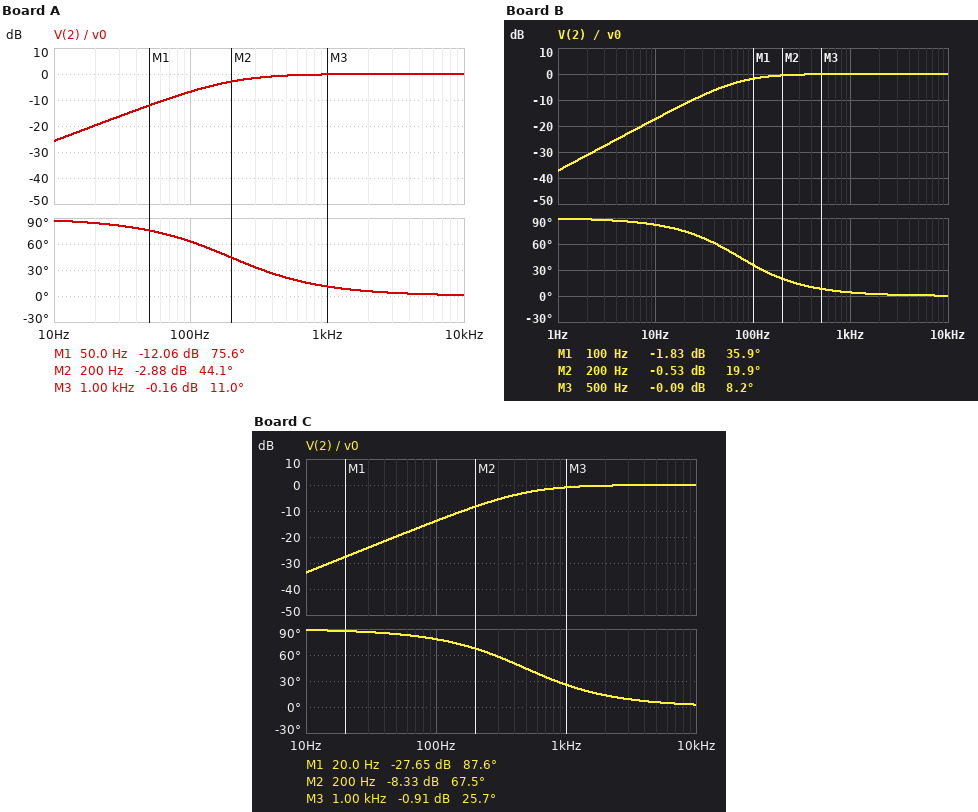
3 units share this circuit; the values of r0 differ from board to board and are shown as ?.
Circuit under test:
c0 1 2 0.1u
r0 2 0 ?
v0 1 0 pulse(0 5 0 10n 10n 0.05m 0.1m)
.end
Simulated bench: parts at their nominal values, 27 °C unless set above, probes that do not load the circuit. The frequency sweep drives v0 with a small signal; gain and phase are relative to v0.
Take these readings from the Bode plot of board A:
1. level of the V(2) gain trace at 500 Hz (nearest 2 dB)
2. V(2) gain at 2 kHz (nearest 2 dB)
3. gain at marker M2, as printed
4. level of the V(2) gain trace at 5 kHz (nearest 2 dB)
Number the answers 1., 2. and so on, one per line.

1. 0 dB
2. 0 dB
3. -2.88 dB
4. 0 dB
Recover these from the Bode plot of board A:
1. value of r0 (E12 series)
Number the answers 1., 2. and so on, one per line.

1. 8.2 kΩ
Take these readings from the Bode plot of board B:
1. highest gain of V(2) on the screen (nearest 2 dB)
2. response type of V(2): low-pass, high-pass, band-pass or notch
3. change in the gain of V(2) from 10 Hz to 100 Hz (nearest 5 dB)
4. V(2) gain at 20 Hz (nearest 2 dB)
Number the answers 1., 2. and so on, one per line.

1. 0 dB
2. high-pass
3. 15 dB
4. -12 dB
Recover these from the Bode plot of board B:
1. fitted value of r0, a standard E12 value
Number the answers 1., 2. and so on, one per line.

1. 22 kΩ
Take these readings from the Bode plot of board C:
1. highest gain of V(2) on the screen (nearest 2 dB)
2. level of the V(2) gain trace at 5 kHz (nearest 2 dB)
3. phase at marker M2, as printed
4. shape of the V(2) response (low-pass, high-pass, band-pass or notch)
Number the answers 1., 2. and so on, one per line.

1. 0 dB
2. 0 dB
3. 67.5 deg
4. high-pass
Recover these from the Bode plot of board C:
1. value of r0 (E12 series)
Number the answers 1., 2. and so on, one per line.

1. 3.3 kΩ
